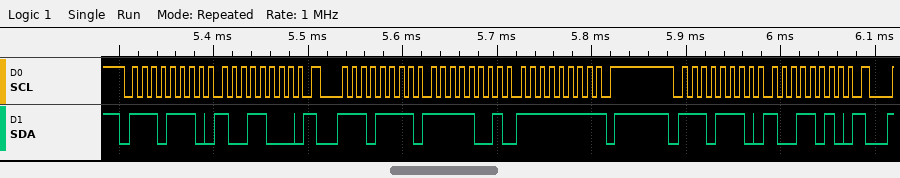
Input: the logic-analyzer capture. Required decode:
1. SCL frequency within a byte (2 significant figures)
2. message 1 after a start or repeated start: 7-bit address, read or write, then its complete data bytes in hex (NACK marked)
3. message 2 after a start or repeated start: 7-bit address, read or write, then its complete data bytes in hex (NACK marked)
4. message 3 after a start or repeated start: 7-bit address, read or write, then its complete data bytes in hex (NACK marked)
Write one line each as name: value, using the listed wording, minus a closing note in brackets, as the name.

SCL frequency within a byte: 100 kHz
message 1 after a start or repeated start: 7-bit address, read or write, then its complete data bytes in hex: 0x77 write: 98
message 2 after a start or repeated start: 7-bit address, read or write, then its complete data bytes in hex: 0x77 read: F9 FF NACK
message 3 after a start or repeated start: 7-bit address, read or write, then its complete data bytes in hex: 0x77 write: 9A
